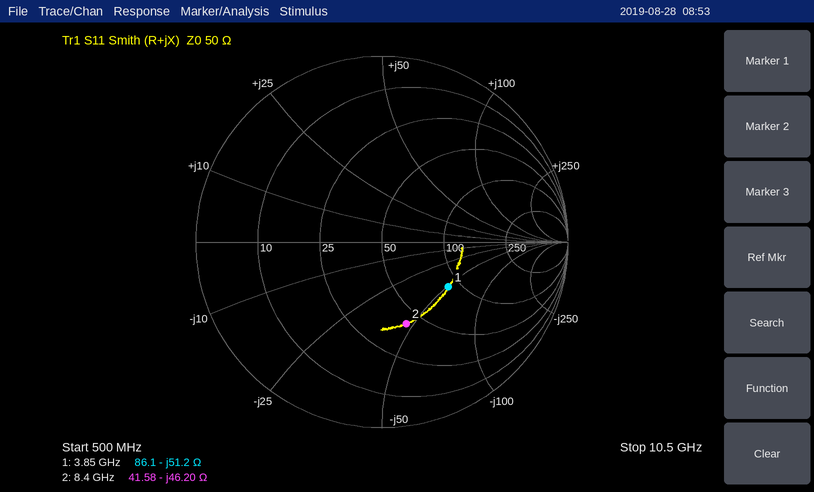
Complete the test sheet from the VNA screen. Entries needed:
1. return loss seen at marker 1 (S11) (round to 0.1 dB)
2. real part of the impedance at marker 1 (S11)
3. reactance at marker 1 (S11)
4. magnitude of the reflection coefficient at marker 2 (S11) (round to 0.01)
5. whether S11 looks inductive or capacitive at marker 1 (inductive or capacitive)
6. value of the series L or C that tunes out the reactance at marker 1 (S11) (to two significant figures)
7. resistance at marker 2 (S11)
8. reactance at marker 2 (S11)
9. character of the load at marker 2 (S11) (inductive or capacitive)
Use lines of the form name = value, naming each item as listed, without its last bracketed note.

return loss seen at marker 1 (S11) = 7.3 dB
real part of the impedance at marker 1 = 86.1 Ω
reactance at marker 1 = -51.2 Ω
magnitude of the reflection coefficient at marker 2 (S11) = 0.46
whether S11 looks inductive or capacitive at marker 1 = capacitive
value of the series L or C that tunes out the reactance at marker 1 (S11) = 2.1 nH
resistance at marker 2 = 41.58 Ω
reactance at marker 2 = -46.20 Ω
character of the load at marker 2 (S11) = capacitive
